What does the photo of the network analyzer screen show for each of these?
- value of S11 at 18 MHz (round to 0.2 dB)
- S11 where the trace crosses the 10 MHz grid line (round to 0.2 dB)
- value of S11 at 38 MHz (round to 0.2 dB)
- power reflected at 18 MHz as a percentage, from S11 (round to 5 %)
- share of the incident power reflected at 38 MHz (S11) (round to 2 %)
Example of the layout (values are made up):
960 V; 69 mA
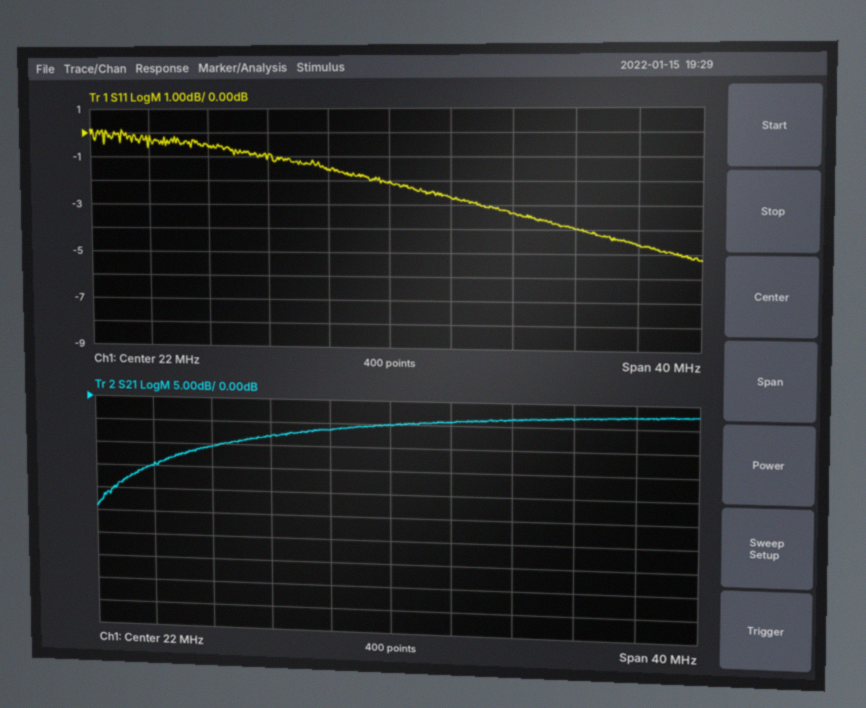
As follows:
-1.6 dB; -0.6 dB; -4.6 dB; 70 %; 34 %
